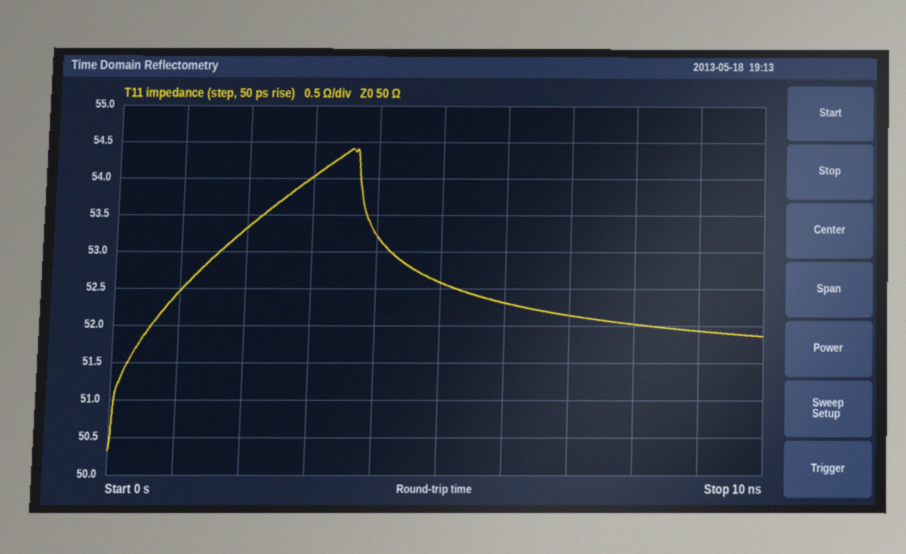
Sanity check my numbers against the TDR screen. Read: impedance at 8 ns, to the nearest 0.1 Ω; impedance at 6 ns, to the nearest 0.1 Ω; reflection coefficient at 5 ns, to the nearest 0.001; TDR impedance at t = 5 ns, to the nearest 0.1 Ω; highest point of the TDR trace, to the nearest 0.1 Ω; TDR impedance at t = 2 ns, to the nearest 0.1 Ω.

52.0 Ω
52.3 Ω
+0.025
52.6 Ω
54.4 Ω
53.3 Ω
